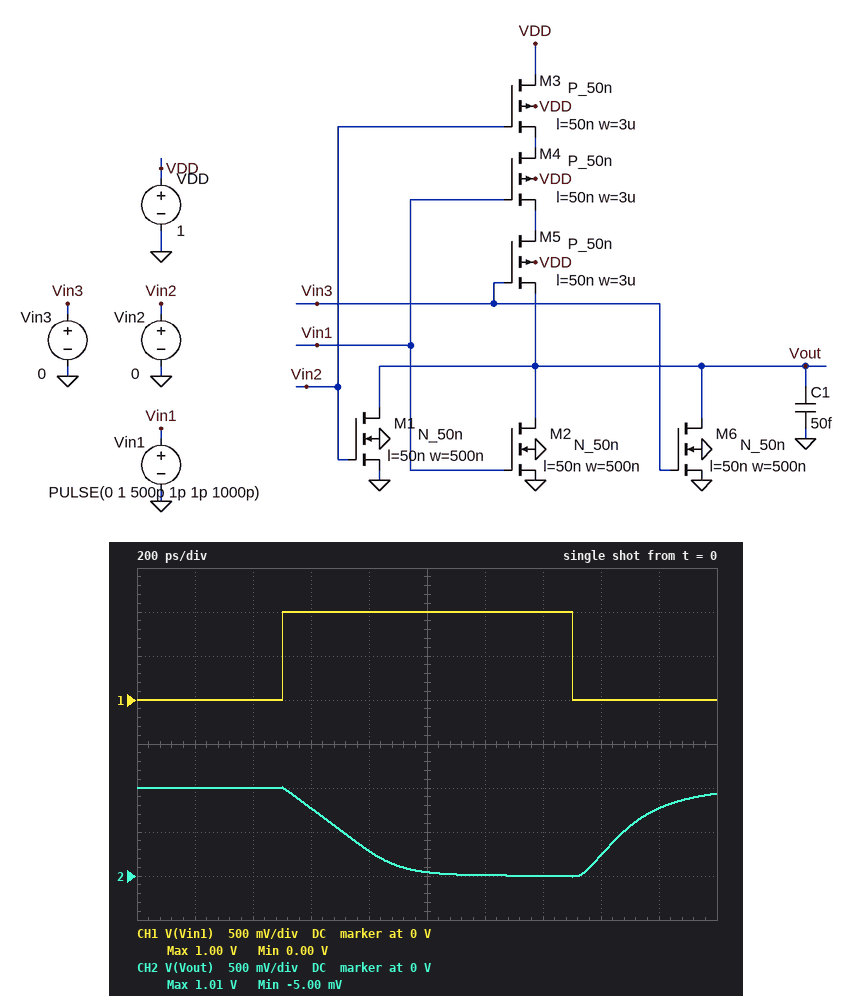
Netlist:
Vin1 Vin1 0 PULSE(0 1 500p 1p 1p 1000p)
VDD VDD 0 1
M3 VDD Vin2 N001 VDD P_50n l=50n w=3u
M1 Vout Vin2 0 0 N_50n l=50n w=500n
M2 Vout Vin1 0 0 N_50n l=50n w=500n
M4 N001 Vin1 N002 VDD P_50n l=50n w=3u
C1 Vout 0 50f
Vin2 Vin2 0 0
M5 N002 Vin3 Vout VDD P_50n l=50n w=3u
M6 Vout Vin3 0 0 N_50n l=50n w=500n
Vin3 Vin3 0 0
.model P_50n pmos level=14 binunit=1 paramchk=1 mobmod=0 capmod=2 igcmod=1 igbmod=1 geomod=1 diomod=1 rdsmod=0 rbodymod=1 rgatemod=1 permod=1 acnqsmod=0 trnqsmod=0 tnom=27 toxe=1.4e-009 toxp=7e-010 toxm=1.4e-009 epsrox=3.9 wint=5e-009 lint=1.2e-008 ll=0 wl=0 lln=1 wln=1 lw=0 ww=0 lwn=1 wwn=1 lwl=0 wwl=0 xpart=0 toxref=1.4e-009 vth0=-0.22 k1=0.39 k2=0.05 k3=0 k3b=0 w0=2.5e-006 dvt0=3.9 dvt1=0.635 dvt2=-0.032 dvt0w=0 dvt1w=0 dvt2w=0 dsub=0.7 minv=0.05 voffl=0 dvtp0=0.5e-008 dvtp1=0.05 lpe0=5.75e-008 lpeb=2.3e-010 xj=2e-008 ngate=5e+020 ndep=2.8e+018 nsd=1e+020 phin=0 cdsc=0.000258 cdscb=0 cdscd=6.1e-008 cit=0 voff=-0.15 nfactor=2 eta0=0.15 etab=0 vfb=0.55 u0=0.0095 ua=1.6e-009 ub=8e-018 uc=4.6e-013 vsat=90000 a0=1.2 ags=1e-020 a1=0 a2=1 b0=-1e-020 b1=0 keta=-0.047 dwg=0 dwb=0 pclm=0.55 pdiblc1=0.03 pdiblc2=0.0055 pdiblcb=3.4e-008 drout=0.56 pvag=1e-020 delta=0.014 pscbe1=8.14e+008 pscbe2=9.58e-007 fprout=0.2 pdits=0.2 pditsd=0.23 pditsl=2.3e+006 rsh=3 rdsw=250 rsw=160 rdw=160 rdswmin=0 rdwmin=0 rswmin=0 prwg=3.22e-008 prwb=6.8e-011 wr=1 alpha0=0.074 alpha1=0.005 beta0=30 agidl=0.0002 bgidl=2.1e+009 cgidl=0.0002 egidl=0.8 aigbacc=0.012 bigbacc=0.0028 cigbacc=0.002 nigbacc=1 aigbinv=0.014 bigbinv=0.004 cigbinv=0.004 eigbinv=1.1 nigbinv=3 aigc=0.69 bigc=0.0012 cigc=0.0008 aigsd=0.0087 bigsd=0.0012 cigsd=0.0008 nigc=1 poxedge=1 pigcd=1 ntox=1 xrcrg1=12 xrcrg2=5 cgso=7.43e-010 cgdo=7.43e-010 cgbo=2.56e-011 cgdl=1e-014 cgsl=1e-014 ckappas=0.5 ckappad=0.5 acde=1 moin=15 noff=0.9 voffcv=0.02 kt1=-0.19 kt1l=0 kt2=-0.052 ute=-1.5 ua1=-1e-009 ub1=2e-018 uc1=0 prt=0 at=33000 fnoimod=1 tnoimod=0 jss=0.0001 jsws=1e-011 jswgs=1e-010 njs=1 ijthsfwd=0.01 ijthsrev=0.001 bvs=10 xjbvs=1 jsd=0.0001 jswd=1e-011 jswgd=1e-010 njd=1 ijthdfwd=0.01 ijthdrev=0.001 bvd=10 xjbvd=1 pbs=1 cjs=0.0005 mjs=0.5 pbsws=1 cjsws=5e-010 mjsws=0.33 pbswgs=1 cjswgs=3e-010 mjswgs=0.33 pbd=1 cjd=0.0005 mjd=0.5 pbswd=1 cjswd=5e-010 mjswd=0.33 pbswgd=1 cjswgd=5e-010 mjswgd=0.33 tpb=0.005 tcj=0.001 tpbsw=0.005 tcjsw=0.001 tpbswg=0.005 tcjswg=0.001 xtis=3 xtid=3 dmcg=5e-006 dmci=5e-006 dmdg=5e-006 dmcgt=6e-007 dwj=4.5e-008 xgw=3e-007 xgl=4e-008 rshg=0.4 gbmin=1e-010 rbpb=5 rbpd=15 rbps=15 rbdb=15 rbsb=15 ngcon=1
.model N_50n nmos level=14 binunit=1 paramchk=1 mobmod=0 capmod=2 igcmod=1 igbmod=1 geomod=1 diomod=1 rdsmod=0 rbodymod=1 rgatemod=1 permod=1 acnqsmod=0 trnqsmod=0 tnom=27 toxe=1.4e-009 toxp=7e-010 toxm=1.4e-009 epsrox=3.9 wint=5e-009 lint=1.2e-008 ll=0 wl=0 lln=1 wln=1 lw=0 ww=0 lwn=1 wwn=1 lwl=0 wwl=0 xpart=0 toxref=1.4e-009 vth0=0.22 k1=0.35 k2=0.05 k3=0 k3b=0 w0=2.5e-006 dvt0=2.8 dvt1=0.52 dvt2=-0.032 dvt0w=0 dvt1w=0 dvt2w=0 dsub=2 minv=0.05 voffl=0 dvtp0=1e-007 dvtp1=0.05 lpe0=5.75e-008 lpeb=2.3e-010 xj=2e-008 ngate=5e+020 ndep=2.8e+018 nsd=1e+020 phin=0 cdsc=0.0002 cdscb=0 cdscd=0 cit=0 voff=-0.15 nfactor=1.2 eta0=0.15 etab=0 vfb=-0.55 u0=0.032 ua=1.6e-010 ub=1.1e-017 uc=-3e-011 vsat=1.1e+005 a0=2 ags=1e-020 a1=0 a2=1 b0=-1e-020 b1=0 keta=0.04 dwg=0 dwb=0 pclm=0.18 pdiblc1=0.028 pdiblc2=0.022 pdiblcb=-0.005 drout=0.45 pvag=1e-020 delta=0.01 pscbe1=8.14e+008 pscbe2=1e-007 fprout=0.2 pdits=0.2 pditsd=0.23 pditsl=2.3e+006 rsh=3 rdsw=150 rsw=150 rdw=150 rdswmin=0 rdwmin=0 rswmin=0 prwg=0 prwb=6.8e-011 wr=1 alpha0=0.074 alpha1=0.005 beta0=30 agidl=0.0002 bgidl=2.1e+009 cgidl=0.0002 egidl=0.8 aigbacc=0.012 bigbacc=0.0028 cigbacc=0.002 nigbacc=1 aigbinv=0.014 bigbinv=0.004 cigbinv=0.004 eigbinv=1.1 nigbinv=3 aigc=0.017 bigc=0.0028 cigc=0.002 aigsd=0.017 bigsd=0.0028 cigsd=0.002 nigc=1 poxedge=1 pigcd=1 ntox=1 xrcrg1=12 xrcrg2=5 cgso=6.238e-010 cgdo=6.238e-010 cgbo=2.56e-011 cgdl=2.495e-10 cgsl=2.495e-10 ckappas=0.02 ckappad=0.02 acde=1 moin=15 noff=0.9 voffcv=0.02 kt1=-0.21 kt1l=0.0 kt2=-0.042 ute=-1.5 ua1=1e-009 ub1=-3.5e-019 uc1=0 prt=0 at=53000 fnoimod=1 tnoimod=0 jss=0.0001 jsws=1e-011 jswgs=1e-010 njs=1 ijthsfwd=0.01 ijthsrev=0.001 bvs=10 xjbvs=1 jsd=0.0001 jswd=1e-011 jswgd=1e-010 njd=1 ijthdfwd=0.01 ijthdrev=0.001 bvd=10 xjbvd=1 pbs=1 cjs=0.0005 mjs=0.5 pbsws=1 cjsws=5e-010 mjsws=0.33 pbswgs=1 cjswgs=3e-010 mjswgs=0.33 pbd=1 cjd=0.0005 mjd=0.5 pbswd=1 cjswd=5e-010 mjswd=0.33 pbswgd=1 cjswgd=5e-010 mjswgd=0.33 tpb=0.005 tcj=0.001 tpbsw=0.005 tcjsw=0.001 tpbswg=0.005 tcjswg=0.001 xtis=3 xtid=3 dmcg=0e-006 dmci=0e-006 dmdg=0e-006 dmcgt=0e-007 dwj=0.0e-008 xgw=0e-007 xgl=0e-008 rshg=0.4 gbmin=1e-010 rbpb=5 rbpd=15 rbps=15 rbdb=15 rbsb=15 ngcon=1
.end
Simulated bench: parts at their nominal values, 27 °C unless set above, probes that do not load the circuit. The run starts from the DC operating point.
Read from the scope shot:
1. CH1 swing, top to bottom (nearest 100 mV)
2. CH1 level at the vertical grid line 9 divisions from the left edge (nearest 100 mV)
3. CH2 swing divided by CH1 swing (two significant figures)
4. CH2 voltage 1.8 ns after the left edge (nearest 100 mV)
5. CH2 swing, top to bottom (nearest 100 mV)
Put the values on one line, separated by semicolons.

1.0 V; 0 V; 1.0; 800 mV; 1.0 V
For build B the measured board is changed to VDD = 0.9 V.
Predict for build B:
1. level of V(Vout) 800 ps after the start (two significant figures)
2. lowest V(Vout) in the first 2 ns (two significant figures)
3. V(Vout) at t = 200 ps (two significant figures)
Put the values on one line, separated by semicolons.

210 mV; -6.4 mV; 900 mV
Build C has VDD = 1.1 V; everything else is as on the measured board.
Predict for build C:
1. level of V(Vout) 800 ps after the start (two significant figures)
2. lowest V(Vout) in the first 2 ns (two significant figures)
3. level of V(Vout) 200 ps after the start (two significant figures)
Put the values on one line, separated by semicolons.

370 mV; -6.1 mV; 1.1 V
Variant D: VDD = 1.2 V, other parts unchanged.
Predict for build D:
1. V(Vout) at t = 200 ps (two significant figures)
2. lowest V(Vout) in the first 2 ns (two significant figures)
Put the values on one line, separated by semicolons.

1.2 V; -4.7 mV
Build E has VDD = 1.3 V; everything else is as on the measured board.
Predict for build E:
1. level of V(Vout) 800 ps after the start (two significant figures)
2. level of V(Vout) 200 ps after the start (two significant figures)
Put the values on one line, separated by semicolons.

560 mV; 1.3 V
